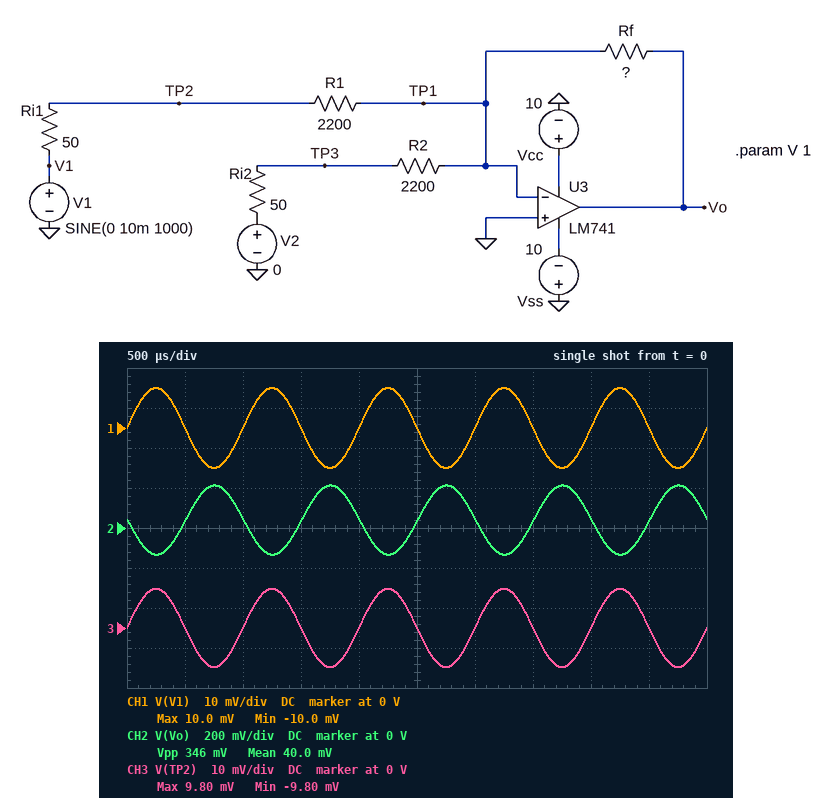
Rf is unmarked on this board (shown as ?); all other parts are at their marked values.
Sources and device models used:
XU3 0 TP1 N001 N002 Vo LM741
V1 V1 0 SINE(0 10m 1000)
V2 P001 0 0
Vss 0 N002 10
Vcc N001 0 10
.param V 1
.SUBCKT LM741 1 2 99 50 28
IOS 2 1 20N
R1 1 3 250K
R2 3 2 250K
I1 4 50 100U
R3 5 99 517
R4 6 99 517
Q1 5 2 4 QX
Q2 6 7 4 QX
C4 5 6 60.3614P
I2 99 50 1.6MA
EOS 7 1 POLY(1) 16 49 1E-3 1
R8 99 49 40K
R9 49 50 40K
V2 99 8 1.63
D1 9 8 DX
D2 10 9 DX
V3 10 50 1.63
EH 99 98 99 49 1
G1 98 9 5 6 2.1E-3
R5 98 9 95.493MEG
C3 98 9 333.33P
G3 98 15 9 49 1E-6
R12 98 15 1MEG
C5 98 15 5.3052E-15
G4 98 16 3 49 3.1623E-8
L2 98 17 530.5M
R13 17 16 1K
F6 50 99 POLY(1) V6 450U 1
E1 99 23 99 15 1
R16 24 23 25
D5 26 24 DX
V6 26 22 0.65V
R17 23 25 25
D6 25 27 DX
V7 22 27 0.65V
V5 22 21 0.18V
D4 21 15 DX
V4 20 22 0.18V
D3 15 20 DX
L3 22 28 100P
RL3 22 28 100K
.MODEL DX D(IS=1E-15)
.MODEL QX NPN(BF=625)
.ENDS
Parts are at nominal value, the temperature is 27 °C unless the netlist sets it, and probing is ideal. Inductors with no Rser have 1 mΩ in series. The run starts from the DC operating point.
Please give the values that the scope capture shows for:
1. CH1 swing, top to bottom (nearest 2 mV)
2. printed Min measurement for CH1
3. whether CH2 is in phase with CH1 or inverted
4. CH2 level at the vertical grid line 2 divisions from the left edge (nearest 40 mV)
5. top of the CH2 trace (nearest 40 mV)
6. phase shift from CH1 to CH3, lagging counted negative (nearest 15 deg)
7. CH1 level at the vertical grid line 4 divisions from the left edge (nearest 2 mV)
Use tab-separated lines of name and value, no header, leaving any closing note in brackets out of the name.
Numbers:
CH1 swing, top to bottom	20 mV
printed Min measurement for CH1	-10.0 mV
whether CH2 is in phase with CH1 or inverted	inverted
CH2 level at the vertical grid line 2 divisions from the left edge	40 mV
top of the CH2 trace	200 mV
phase shift from CH1 to CH3, lagging counted negative	0 deg
CH1 level at the vertical grid line 4 divisions from the left edge	0 V
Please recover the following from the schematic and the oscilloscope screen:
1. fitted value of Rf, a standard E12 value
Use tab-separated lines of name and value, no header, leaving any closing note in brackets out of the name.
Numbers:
fitted value of Rf, a standard E12 value	39 kΩ
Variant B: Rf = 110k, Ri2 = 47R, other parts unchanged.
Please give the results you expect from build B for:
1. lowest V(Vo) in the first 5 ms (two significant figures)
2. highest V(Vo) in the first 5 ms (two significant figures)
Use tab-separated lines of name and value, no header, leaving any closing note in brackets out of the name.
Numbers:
lowest V(Vo) in the first 5 ms	-380 mV
highest V(Vo) in the first 5 ms	600 mV
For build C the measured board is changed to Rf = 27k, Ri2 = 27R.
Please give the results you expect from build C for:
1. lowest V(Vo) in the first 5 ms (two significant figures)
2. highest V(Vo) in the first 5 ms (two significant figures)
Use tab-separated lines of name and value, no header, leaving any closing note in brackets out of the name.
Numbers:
lowest V(Vo) in the first 5 ms	-92 mV
highest V(Vo) in the first 5 ms	150 mV
